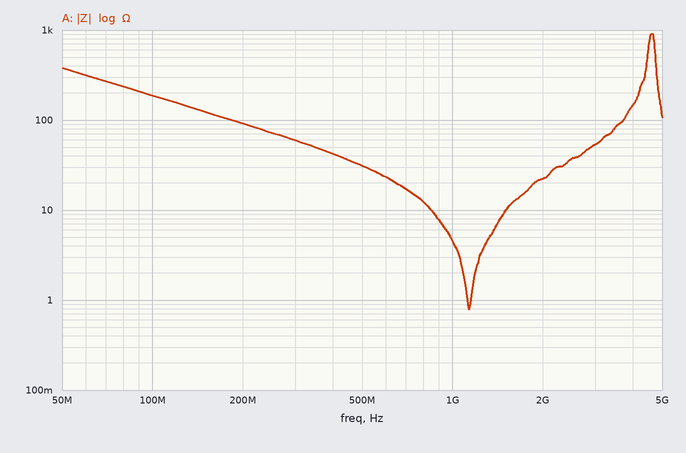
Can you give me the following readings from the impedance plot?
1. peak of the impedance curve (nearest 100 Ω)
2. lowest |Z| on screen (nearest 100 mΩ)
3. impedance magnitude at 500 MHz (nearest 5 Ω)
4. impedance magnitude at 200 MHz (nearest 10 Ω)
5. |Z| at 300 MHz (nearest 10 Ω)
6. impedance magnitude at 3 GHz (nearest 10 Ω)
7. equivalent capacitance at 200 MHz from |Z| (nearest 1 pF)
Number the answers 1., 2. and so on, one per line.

1. 900 Ω
2. 800 mΩ
3. 30 Ω
4. 90 Ω
5. 60 Ω
6. 50 Ω
7. 9 pF
